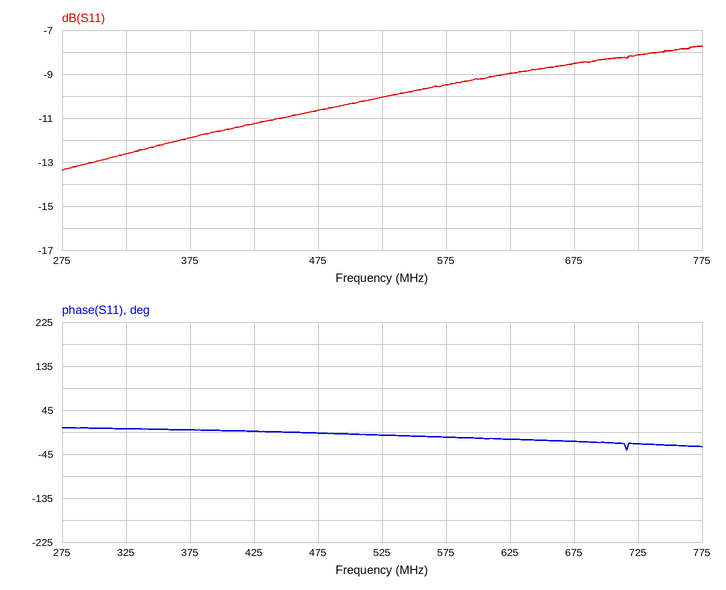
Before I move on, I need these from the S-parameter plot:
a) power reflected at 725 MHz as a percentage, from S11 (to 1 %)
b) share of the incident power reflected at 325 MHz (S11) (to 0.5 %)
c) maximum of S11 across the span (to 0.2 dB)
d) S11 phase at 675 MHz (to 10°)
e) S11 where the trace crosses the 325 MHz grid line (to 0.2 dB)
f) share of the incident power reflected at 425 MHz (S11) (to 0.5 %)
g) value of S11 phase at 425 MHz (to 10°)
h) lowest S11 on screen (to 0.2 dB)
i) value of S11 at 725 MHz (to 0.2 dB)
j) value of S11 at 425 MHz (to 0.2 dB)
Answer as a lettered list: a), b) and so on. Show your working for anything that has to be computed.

a) 10^(-8.2/10) ≈ 15 %
b) 10^(-12.6/10) ≈ 5.5 %
c) -7.8 dB
d) -20°
e) -12.6 dB
f) 10^(-11.2/10) ≈ 7.59 %, so 7.5 % to the nearest 0.5 %
g) 0°
h) -13.4 dB
i) -8.2 dB
j) -11.2 dB
